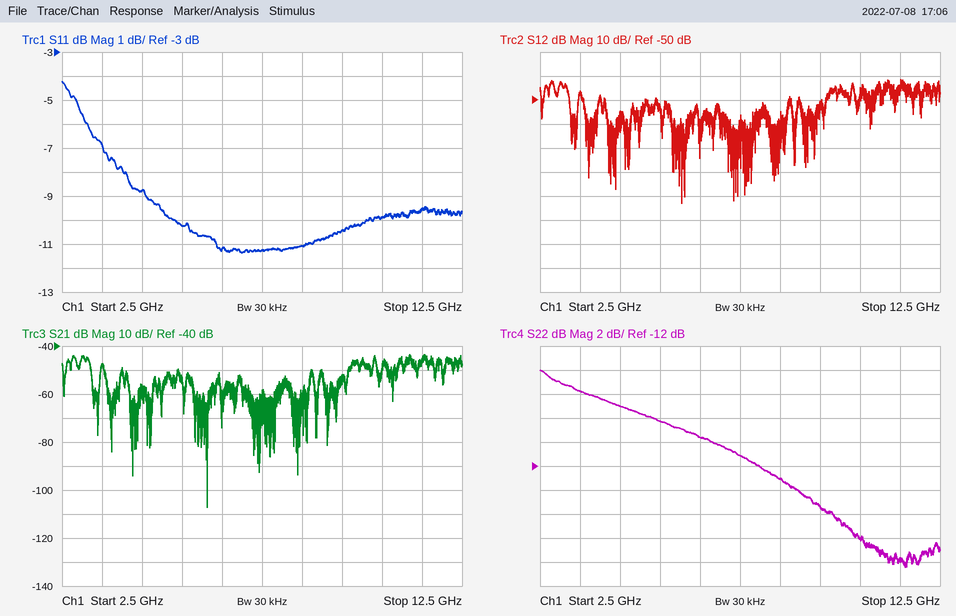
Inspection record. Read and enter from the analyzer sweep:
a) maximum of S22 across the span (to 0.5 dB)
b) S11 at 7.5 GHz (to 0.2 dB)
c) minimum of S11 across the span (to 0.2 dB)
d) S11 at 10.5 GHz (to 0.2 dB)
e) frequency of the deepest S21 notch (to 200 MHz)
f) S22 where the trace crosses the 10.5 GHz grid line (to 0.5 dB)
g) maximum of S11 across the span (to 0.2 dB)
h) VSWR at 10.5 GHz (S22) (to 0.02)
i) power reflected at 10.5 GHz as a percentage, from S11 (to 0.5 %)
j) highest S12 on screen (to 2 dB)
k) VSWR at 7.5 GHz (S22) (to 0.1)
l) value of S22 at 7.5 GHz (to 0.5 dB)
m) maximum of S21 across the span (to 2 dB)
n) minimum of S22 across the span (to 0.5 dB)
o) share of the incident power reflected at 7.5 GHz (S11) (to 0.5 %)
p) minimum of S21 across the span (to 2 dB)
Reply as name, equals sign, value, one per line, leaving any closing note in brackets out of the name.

maximum of S22 across the span = -4.0 dB
S11 at 7.5 GHz = -11.2 dB
minimum of S11 across the span = -11.4 dB
S11 at 10.5 GHz = -9.8 dB
frequency of the deepest S21 notch = 6.2 GHz
S22 where the trace crosses the 10.5 GHz grid line = -18.0 dB
maximum of S11 across the span = -4.2 dB
VSWR at 10.5 GHz (S22) = 1.28
power reflected at 10.5 GHz as a percentage, from S11 = 10.5 %
highest S12 on screen = -42 dB
VSWR at 7.5 GHz (S22) = 1.8
value of S22 at 7.5 GHz = -11.0 dB
maximum of S21 across the span = -44 dB
minimum of S22 across the span = -20.5 dB
share of the incident power reflected at 7.5 GHz (S11) = 7.5 %
minimum of S21 across the span = -108 dB
